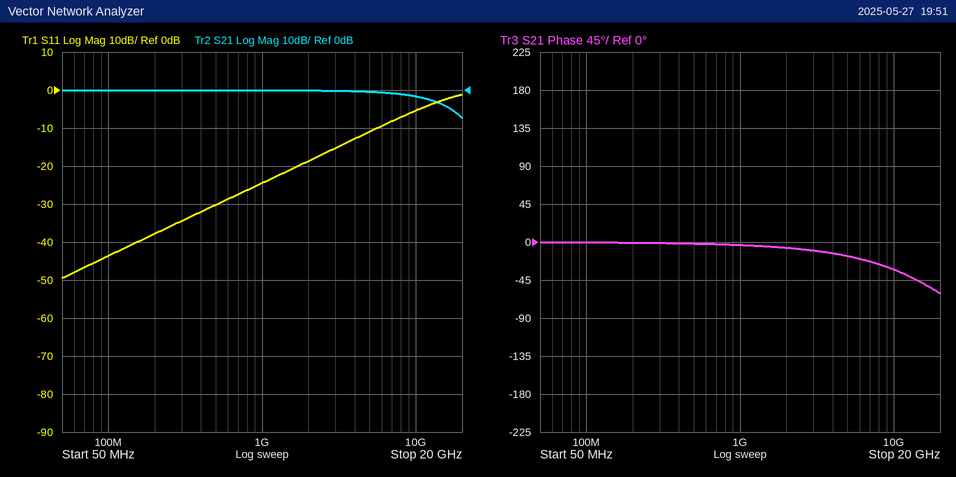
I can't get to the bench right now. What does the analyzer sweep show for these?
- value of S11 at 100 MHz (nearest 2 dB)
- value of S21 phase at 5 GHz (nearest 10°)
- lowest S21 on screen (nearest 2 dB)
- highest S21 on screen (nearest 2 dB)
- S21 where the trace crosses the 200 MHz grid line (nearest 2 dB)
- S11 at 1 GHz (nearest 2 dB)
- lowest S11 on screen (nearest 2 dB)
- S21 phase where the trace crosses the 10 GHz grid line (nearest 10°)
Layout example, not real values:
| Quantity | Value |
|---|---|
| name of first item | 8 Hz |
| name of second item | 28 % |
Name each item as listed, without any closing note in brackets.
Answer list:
| Quantity | Value |
|---|---|
| value of S11 at 100 MHz | -44 dB |
| value of S21 phase at 5 GHz | -20° |
| lowest S21 on screen | -8 dB |
| highest S21 on screen | 0 dB |
| S21 where the trace crosses the 200 MHz grid line | 0 dB |
| S11 at 1 GHz | -24 dB |
| lowest S11 on screen | -50 dB |
| S21 phase where the trace crosses the 10 GHz grid line | -30° |
